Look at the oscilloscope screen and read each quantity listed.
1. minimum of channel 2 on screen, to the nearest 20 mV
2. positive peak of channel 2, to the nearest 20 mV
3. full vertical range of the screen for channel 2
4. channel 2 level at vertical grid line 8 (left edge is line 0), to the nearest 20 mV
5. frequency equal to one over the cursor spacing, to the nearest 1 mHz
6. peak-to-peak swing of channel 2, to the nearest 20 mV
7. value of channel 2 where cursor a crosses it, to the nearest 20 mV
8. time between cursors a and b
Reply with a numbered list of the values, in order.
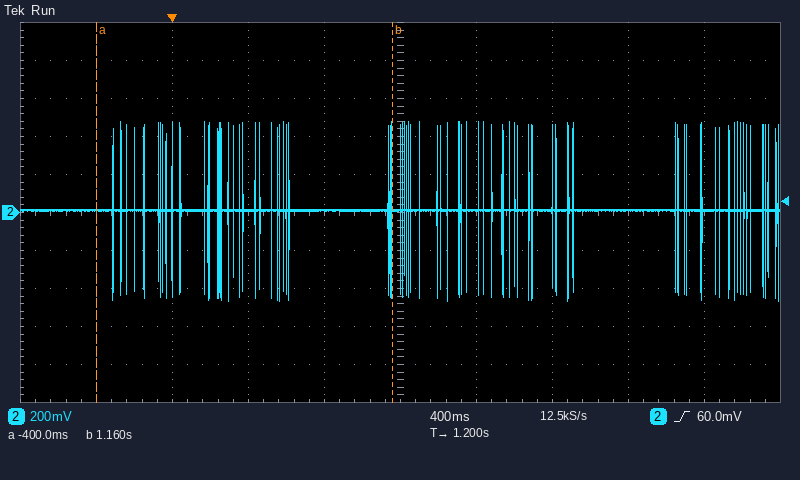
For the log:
1. -460 mV
2. 480 mV
3. 2 V
4. 20 mV
5. 641 mHz
6. 940 mV
7. 20 mV
8. 1.56 s
